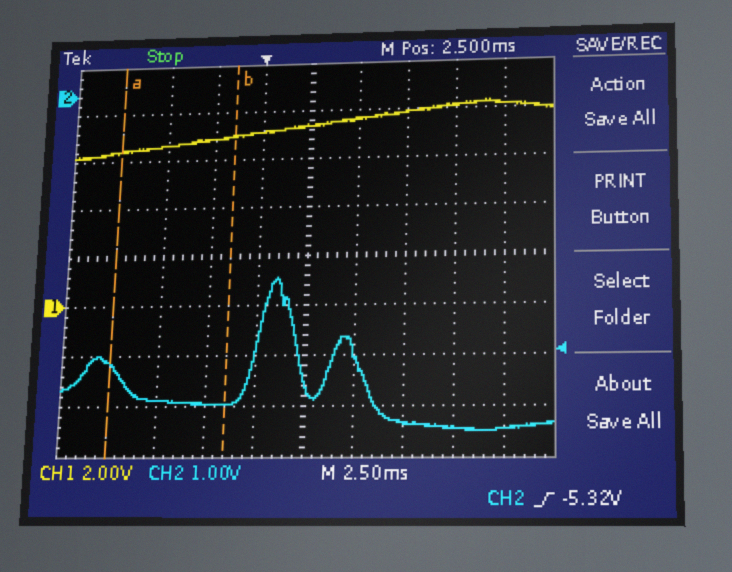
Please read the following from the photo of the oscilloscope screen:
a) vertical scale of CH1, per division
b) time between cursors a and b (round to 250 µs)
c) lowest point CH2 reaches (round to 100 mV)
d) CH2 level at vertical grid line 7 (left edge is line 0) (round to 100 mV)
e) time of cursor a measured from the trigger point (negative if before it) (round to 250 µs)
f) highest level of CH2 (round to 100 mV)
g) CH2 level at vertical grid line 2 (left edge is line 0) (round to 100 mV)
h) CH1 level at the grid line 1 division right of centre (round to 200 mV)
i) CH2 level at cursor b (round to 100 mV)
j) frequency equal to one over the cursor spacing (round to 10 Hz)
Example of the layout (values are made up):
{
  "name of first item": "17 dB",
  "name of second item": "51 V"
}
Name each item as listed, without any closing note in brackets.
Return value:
{
  "vertical scale of CH1, per division": "2 V",
  "time between cursors a and b": "6.00 ms",
  "lowest point CH2 reaches": "-6.9 V",
  "CH2 level at vertical grid line 7 (left edge is line 0)": "-6.7 V",
  "time of cursor a measured from the trigger point (negative if before it)": "-7.50 ms",
  "highest level of CH2": "-3.8 V",
  "CH2 level at vertical grid line 2 (left edge is line 0)": "-6.3 V",
  "CH1 level at the grid line 1 division right of centre": "7.6 V",
  "CH2 level at cursor b": "-6.4 V",
  "frequency equal to one over the cursor spacing": "170 Hz"
}
